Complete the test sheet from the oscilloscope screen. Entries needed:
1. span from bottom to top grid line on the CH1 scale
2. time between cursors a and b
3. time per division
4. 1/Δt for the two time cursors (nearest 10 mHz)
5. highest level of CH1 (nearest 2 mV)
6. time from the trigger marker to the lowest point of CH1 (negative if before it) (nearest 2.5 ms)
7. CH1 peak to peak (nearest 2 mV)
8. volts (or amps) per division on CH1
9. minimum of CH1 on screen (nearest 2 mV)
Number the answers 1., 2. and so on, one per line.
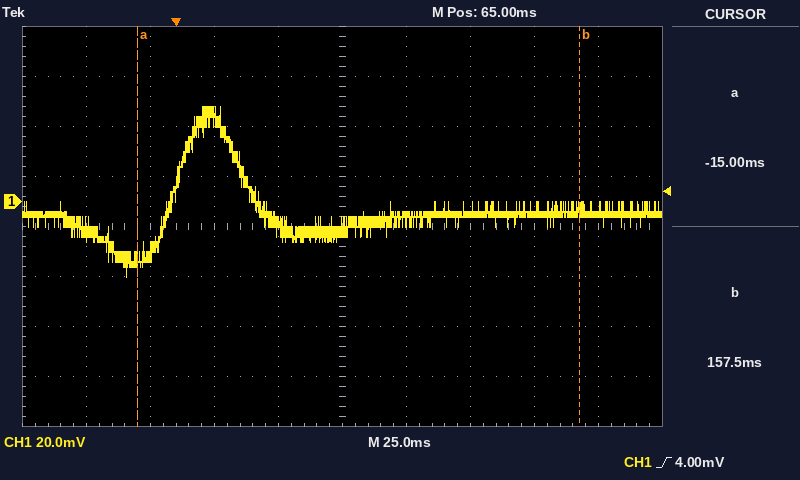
1. 160 mV
2. 172.5 ms
3. 25 ms
4. 5.80 Hz
5. 38 mV
6. -20.0 ms
7. 68 mV
8. 20 mV
9. -30 mV
